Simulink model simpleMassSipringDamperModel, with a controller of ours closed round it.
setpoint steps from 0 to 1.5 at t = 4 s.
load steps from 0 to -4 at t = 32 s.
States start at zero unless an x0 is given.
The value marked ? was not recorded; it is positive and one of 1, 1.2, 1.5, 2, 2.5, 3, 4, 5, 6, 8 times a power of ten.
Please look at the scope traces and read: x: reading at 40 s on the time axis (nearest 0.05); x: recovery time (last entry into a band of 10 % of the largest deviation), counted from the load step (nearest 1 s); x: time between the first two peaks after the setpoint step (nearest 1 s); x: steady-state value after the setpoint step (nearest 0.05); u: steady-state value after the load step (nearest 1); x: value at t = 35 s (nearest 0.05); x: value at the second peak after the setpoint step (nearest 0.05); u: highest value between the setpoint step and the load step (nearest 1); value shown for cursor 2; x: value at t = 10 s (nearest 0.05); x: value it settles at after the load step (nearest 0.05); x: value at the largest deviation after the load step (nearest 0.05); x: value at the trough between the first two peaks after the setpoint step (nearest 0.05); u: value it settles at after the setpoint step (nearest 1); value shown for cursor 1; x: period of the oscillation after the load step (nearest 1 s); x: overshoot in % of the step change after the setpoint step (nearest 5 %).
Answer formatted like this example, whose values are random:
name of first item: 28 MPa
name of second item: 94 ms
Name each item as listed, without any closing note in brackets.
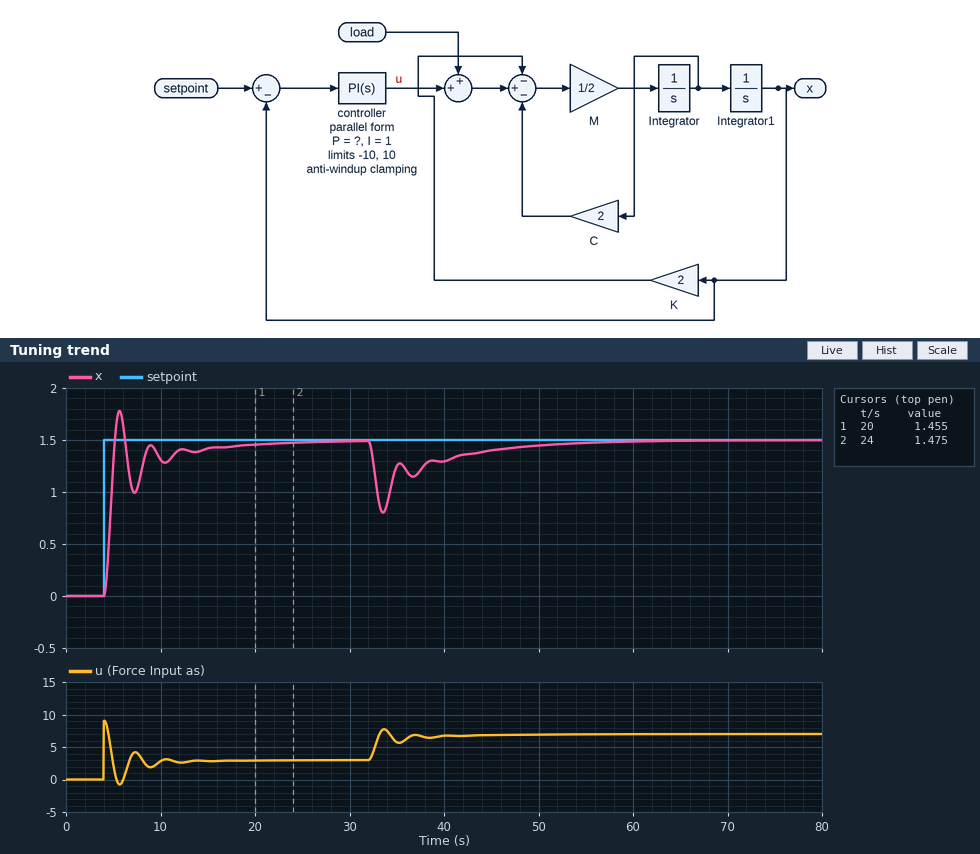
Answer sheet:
x: reading at 40 s on the time axis: 1.30
x: recovery time (last entry into a band of 10 % of the largest deviation), counted from the load step: 16 s
x: time between the first two peaks after the setpoint step: 3 s
x: steady-state value after the setpoint step: 1.50
u: steady-state value after the load step: 7
x: value at t = 35 s: 1.25
x: value at the second peak after the setpoint step: 1.45
u: highest value between the setpoint step and the load step: 9
value shown for cursor 2: 1.475
x: value at t = 10 s: 1.30
x: value it settles at after the load step: 1.50
x: value at the largest deviation after the load step: 0.80
x: value at the trough between the first two peaks after the setpoint step: 1.00
u: value it settles at after the setpoint step: 3
value shown for cursor 1: 1.455
x: period of the oscillation after the load step: 3 s
x: overshoot in % of the step change after the setpoint step: 20 %
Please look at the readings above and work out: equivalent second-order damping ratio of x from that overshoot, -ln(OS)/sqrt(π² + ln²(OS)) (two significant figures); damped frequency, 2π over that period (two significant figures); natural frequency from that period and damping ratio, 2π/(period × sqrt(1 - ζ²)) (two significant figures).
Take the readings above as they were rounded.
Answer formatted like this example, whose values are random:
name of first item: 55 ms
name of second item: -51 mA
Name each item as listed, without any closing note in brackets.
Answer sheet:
equivalent second-order damping ratio of x from that overshoot, -ln(OS)/sqrt(π² + ln²(OS)): 0.46
damped frequency, 2π over that period: 2.1 rad/s
natural frequency from that period and damping ratio, 2π/(period × sqrt(1 - ζ²)): 2.4 rad/s
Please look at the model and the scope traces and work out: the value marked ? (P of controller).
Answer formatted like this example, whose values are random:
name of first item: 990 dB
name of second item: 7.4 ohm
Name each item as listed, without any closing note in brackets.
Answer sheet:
the value marked ?: 6
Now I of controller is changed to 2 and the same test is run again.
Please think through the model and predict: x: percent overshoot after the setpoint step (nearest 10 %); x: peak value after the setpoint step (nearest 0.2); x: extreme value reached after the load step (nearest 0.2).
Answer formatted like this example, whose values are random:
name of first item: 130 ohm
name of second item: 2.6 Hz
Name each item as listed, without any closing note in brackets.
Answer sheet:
x: percent overshoot after the setpoint step: 30 %
x: peak value after the setpoint step: 2.0
x: extreme value reached after the load step: 0.8
